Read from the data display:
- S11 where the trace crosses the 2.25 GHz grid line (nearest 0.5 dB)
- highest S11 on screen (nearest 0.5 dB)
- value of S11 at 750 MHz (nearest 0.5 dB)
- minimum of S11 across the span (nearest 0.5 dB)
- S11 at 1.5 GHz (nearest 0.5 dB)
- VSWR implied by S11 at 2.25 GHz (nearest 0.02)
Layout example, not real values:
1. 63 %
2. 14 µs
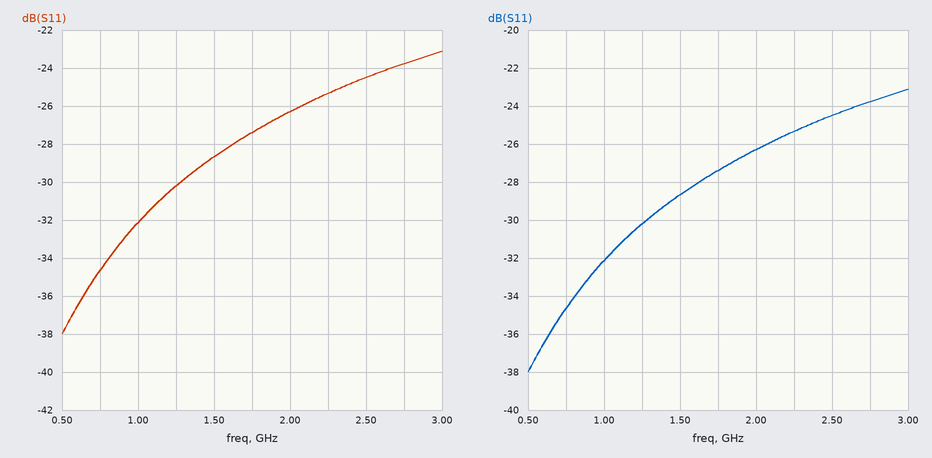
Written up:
1. -25.5 dB
2. -23.0 dB
3. -34.5 dB
4. -38.0 dB
5. -28.5 dB
6. 1.12
